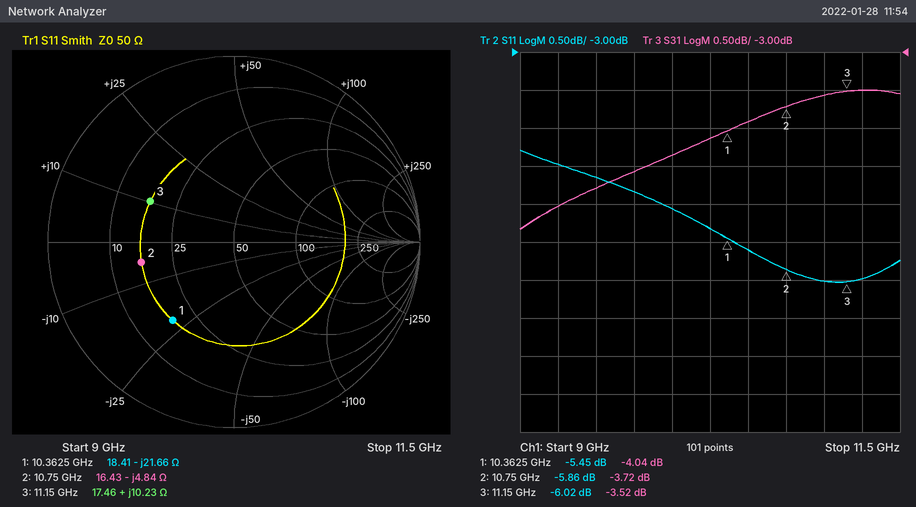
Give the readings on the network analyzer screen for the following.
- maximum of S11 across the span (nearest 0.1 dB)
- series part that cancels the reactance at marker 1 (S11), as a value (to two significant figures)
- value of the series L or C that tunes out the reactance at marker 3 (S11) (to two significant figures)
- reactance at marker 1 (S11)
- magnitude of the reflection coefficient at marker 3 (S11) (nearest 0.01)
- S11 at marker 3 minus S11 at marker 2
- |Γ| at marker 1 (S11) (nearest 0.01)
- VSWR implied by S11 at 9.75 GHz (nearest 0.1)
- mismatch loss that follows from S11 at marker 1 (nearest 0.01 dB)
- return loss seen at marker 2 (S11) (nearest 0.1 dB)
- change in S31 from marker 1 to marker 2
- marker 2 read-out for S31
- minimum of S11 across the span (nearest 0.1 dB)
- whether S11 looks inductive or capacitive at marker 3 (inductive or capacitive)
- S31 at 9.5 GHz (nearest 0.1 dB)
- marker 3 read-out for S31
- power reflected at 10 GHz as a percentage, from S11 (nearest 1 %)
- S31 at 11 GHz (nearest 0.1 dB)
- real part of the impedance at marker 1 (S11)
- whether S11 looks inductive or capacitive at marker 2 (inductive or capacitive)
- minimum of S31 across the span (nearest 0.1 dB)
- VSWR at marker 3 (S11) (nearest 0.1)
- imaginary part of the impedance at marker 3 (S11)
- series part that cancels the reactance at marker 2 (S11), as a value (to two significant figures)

-4.3 dB
330 pH
1.4 pF
-21.66 Ω
0.50
-0.16 dB
0.53
3.7
1.46 dB
5.9 dB
0.32 dB
-3.72 dB
-6.0 dB
inductive
-4.8 dB
-3.52 dB
31 %
-3.6 dB
18.41 Ω
capacitive
-5.3 dB
3.0
+10.23 Ω
72 pH
